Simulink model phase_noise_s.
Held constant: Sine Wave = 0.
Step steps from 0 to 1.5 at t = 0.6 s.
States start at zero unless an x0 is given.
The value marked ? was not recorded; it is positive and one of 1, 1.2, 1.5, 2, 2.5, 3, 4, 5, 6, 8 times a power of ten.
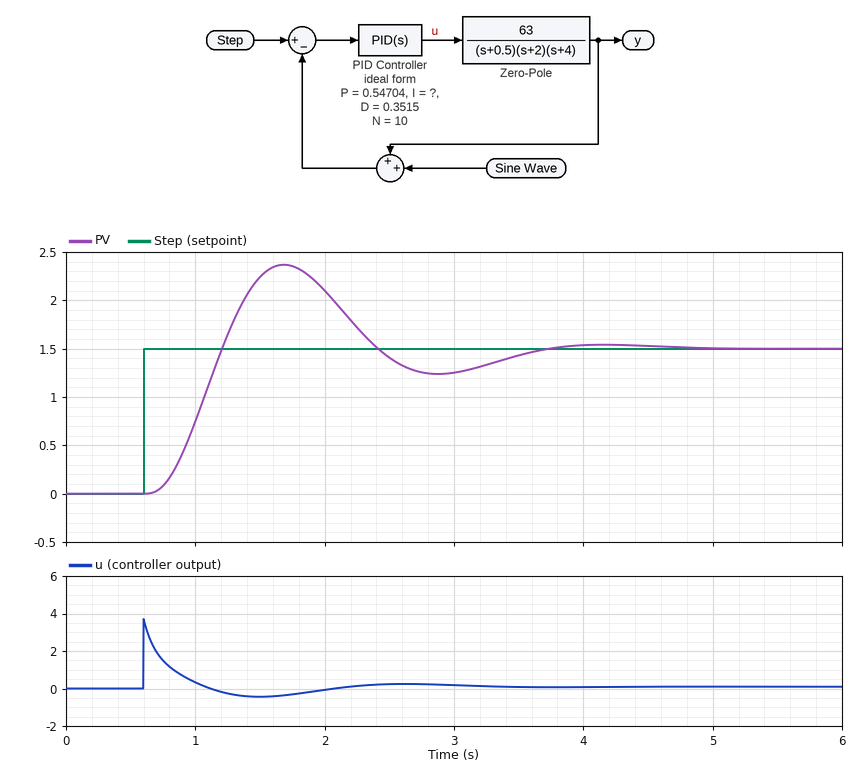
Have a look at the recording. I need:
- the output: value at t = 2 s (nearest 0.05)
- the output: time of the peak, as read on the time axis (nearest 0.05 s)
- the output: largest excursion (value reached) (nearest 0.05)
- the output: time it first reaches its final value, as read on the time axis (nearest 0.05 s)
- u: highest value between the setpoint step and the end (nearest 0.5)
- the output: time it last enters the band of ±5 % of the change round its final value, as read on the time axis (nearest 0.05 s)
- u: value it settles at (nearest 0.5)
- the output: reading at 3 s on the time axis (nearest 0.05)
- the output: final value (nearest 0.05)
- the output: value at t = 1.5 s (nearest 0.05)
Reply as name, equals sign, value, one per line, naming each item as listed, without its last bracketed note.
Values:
the output: value at t = 2 s = 2.10
the output: time of the peak, as read on the time axis = 1.70 s
the output: largest excursion (value reached) = 2.35
the output: time it first reaches its final value, as read on the time axis = 1.20 s
u: highest value between the setpoint step and the end = 3.5
the output: time it last enters the band of ±5 % of the change round its final value, as read on the time axis = 3.50 s
u: value it settles at = 0.0
the output: reading at 3 s on the time axis = 1.25
the output: final value = 1.50
the output: value at t = 1.5 s = 2.25
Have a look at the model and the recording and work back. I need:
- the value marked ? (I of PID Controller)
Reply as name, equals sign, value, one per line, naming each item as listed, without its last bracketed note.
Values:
the value marked ? = 1.5
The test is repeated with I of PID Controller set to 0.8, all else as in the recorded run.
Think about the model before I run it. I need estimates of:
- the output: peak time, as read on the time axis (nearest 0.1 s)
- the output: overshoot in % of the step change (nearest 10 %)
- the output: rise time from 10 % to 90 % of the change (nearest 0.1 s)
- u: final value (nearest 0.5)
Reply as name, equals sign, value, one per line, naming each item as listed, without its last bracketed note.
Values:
the output: peak time, as read on the time axis = 1.6 s
the output: overshoot in % of the step change = 40 %
the output: rise time from 10 % to 90 % of the change = 0.4 s
u: final value = 0.0
